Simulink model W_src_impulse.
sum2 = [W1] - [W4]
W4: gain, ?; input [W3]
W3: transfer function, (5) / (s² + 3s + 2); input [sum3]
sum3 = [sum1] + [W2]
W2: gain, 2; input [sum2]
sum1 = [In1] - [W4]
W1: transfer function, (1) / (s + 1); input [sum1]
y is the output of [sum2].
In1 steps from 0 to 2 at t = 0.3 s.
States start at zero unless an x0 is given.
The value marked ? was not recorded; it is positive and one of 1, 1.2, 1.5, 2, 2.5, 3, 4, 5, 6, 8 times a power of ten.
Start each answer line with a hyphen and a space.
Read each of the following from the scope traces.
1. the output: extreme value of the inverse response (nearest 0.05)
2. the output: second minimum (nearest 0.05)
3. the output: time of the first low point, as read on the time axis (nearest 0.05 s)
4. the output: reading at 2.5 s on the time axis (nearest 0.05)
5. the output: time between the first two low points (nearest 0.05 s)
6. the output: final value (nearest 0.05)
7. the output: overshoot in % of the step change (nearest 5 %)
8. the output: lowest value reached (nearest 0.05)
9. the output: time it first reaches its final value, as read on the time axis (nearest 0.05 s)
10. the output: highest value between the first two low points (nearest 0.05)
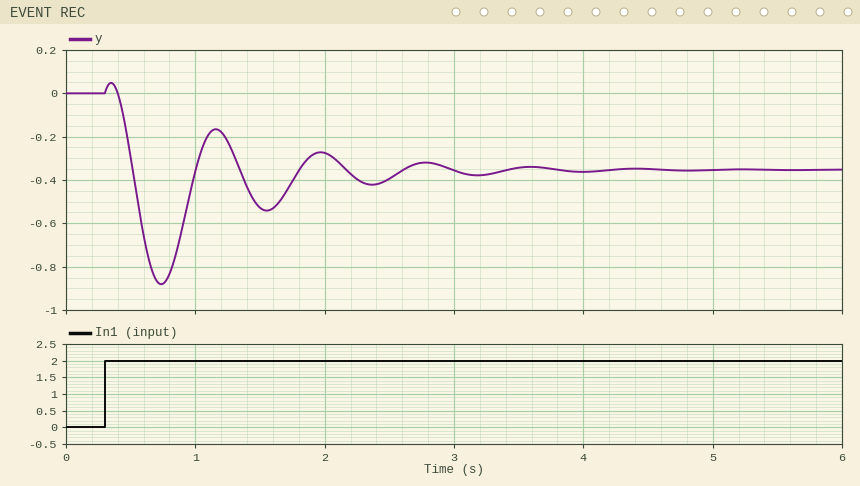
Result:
- 0.05
- -0.55
- 0.75 s
- -0.40
- 0.80 s
- -0.35
- 150 %
- -0.90
- 0.50 s
- -0.15
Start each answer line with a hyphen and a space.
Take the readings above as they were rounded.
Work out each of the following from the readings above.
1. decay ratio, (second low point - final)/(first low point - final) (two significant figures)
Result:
- 0.36
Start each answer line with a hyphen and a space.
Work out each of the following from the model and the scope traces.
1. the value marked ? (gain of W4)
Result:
- 4
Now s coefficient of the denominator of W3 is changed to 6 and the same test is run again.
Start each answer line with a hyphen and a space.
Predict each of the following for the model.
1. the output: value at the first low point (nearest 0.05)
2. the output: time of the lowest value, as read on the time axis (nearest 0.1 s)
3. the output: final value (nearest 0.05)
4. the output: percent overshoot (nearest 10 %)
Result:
- -0.65
- 0.8 s
- -0.35
- 80 %
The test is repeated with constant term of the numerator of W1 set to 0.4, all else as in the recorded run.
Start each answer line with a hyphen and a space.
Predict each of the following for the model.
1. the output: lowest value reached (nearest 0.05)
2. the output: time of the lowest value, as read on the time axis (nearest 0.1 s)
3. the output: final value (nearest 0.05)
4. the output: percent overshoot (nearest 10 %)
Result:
- -0.95
- 0.7 s
- -0.50
- 90 %
